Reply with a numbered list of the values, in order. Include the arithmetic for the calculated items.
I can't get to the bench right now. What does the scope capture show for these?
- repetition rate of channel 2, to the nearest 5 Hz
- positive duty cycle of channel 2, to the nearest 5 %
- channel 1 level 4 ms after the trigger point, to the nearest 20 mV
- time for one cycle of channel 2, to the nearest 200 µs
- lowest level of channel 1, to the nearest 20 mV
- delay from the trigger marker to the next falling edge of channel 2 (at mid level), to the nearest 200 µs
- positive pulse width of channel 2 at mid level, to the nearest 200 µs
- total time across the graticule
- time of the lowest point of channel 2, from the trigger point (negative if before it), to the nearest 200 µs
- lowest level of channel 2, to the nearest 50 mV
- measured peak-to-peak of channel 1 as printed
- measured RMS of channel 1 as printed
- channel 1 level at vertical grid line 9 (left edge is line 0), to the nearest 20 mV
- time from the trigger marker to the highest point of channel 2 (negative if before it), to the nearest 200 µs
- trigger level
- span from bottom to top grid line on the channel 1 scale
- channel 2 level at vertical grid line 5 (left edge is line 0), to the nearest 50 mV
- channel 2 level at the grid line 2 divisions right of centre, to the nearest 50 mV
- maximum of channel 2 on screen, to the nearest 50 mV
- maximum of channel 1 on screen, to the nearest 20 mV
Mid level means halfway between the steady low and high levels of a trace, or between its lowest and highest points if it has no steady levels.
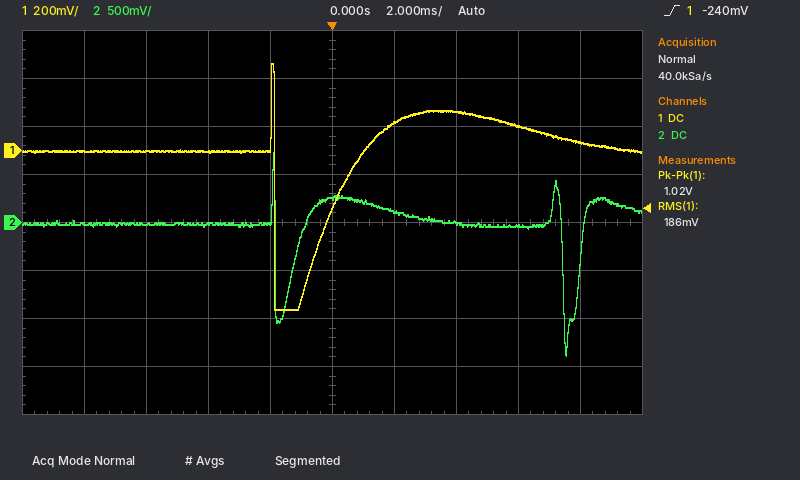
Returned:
1. 1 / 9.2 ms ≈ 109 Hz, so 110 Hz to the nearest 5 Hz
2. 8.6 ms / 9.2 ms ≈ 93.5 %, so 95 % to the nearest 5 %
3. 160 mV
4. 9.2 ms
5. -660 mV
6. 7.4 ms
7. 8.6 ms
8. 20 ms
9. +7.6 ms
10. -1.40 V
11. 1.02 V
12. 186 mV
13. 40 mV
14. -1.8 ms
15. -240 mV
16. 1.6 V
17. 250 mV
18. 0 mV
19. 750 mV
20. 360 mV
